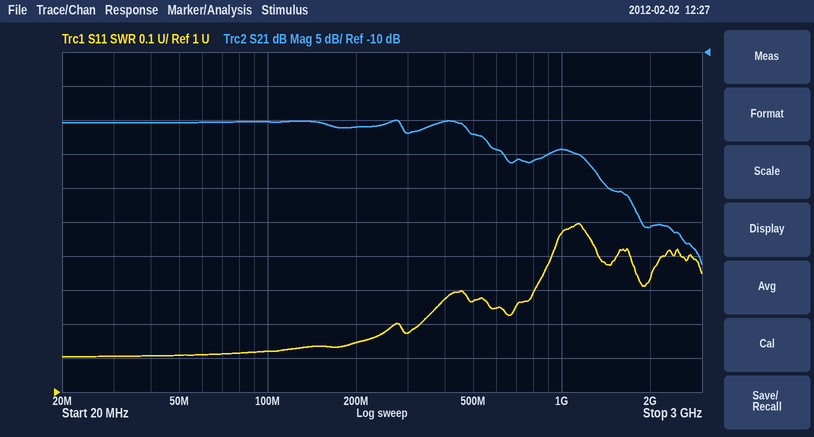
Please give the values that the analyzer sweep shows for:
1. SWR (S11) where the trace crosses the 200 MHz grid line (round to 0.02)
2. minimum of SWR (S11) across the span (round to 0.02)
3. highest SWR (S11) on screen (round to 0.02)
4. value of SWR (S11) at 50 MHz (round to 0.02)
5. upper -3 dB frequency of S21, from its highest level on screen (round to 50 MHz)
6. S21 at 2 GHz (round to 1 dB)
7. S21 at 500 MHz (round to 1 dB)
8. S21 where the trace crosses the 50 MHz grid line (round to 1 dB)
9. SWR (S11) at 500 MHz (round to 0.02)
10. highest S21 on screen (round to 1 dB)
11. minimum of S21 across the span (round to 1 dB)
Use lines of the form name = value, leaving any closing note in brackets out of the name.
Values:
SWR (S11) where the trace crosses the 200 MHz grid line = 1.14
minimum of SWR (S11) across the span = 1.10
highest SWR (S11) on screen = 1.50
value of SWR (S11) at 50 MHz = 1.10
upper -3 dB frequency of S21, from its highest level on screen = 550 MHz
S21 at 2 GHz = -36 dB
S21 at 500 MHz = -22 dB
S21 where the trace crosses the 50 MHz grid line = -20 dB
SWR (S11) at 500 MHz = 1.26
highest S21 on screen = -20 dB
minimum of S21 across the span = -41 dB
